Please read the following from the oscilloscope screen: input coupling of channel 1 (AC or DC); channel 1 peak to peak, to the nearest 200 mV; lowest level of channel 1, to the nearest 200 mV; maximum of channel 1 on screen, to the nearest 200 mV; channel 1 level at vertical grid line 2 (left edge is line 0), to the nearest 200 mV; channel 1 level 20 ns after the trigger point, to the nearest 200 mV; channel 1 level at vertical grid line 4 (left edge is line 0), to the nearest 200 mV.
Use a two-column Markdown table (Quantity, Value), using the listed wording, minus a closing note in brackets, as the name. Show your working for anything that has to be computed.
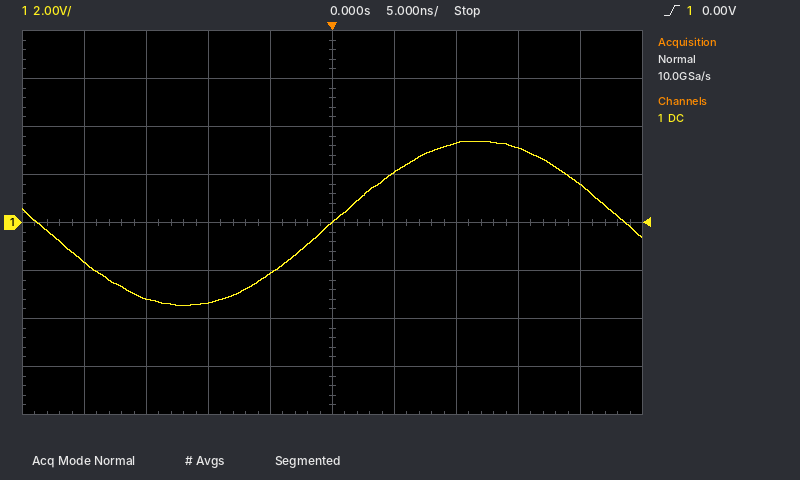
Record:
| Quantity | Value |
|---|---|
| input coupling of channel 1 | DC |
| channel 1 peak to peak, to the nearest 200 mV | 3.4 V − (-3.4 V) = 6.8 V |
| lowest level of channel 1, to the nearest 200 mV | -3.4 V |
| maximum of channel 1 on screen, to the nearest 200 mV | 3.4 V |
| channel 1 level at vertical grid line 2 (left edge is line 0), to the nearest 200 mV | -3.2 V |
| channel 1 level 20 ns after the trigger point, to the nearest 200 mV | 1.6 V |
| channel 1 level at vertical grid line 4 (left edge is line 0), to the nearest 200 mV | -2.2 V |
